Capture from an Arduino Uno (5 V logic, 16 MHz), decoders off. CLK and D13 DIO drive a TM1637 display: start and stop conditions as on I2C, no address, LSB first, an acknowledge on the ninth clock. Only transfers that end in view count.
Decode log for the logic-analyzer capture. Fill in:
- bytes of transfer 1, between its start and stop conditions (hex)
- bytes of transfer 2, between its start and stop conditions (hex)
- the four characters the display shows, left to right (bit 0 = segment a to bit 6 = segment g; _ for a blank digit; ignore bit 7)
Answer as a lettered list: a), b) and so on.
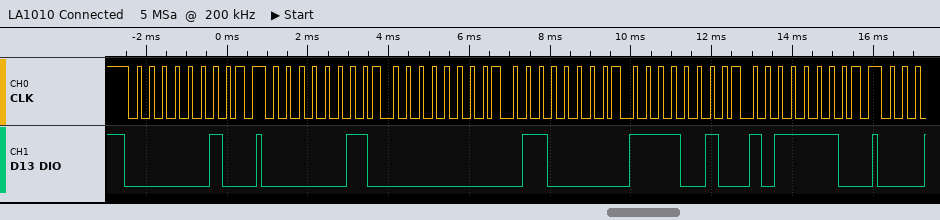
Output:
a) 40
b) C0 00 06 4F 7D
c) _136
